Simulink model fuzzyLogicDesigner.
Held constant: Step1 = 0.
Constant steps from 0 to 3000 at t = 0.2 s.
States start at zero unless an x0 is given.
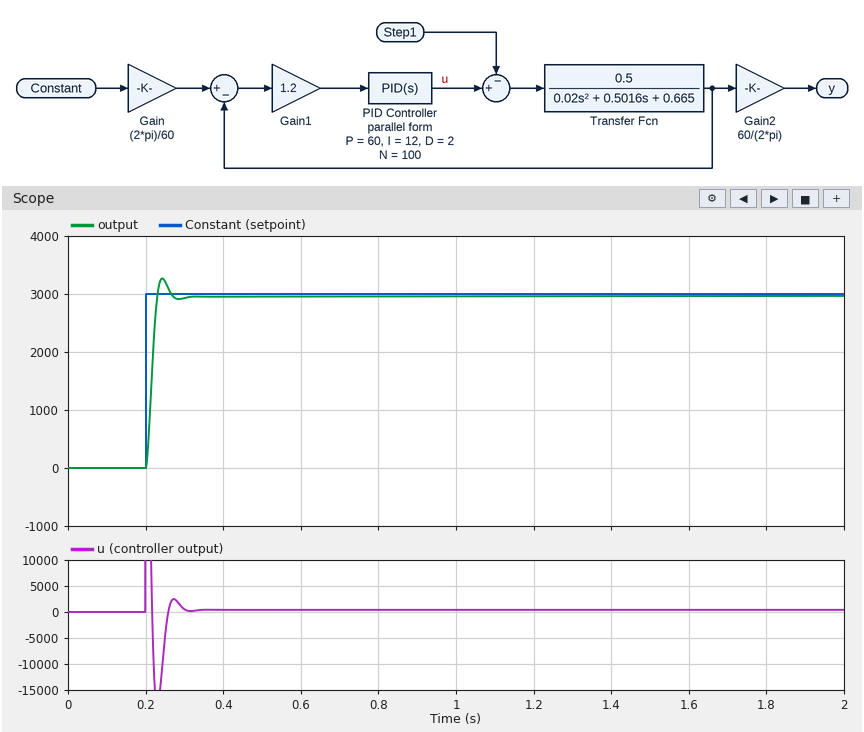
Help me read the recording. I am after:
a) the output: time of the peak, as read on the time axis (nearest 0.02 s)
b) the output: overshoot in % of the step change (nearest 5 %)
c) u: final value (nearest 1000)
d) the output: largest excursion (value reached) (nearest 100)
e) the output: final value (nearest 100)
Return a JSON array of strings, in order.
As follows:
["0.24 s", "10 %", "0", "3300", "3000"]
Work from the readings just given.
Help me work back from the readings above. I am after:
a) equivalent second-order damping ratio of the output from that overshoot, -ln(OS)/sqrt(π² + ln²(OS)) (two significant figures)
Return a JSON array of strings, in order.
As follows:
["0.59"]
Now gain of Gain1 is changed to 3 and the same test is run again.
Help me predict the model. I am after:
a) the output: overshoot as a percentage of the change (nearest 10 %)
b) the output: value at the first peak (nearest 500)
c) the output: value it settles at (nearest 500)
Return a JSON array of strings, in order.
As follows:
["30 %", "4000", "3000"]
